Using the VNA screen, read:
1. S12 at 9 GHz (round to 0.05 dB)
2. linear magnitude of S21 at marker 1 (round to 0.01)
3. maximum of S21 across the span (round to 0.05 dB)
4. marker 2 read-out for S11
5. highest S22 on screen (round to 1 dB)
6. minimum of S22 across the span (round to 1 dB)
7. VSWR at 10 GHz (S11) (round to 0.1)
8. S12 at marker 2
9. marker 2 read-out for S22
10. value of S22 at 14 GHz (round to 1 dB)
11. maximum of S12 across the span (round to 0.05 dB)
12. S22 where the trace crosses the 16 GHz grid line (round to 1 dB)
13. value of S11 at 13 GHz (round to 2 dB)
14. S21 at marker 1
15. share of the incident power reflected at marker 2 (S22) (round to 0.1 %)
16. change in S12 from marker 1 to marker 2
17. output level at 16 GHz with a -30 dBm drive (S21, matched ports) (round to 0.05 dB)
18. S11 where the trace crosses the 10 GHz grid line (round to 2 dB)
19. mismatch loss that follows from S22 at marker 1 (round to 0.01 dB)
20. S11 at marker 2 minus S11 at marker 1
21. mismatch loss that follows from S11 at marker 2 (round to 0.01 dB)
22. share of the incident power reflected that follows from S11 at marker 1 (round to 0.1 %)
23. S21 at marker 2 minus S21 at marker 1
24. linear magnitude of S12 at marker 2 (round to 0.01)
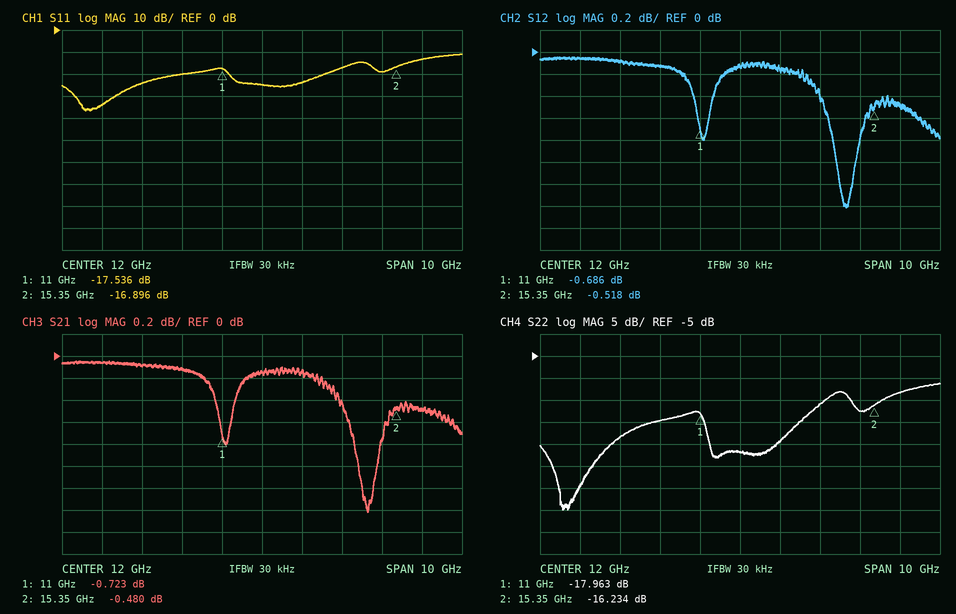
-0.10 dB
0.92
-0.05 dB
-16.896 dB
-11 dB
-40 dB
1.2
-0.518 dB
-16.234 dB
-16 dB
-0.05 dB
-13 dB
-24 dB
-0.723 dB
2.4 %
0.168 dB
-30.50 dBm
-20 dB
0.07 dB
0.640 dB
0.09 dB
1.8 %
0.243 dB
0.94
